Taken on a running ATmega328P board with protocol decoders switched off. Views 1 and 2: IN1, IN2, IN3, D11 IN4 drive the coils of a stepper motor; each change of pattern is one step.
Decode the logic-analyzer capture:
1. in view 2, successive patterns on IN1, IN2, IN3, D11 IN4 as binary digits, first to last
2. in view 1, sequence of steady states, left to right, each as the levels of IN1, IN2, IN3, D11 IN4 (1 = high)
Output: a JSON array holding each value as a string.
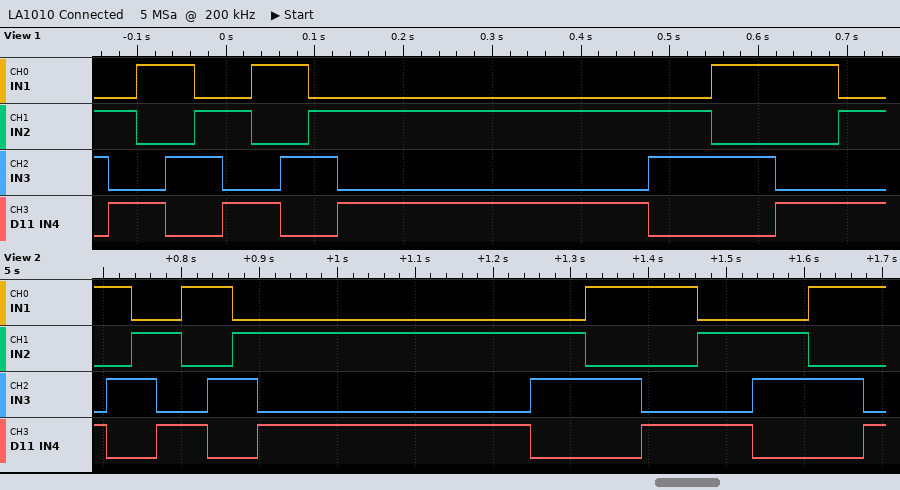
["1001 1010 0110 0101 1001 1010 0110 0101 0110 1010 1001 0101 0110 1010 1001", "0110 0101 1001 1010 0110 0101 1001 1010 0110 0101 0110 1010 1001 0101"]
